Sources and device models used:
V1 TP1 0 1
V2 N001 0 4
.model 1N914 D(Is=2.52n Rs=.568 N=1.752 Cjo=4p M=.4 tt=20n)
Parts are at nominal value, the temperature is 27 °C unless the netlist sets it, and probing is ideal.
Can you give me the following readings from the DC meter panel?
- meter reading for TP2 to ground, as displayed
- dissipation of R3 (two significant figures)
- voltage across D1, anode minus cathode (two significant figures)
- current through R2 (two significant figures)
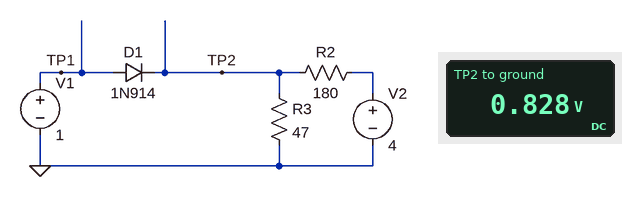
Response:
0.828 V
15 mW
170 mV
18 mA
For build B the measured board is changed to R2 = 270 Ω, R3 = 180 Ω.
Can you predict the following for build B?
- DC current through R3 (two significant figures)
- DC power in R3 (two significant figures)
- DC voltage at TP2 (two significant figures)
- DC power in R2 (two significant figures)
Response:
8.9 mA
14 mW
1.6 V
21 mW
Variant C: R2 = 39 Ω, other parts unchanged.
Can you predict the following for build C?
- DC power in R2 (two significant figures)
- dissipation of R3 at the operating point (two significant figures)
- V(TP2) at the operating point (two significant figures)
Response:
84 mW
100 mW
2.2 V
